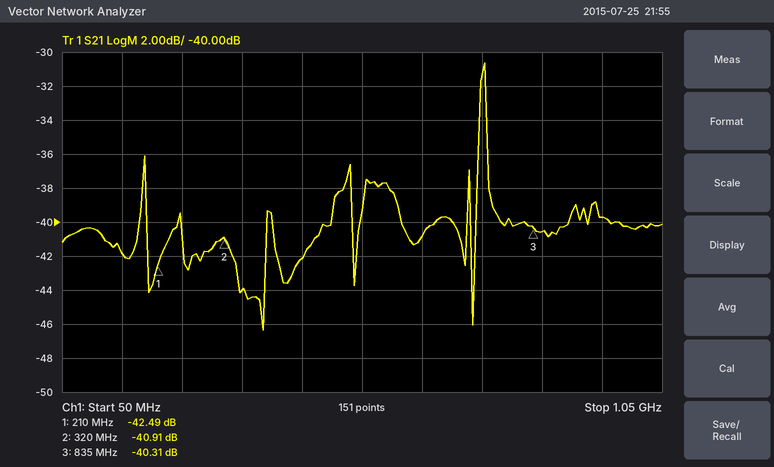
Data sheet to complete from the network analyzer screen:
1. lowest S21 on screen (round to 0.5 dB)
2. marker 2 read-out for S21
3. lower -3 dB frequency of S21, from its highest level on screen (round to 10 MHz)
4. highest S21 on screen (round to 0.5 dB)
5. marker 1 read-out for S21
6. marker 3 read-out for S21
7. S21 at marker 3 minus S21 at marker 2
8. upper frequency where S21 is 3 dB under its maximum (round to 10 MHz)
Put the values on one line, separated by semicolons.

-46.5 dB; -40.91 dB; 750 MHz; -30.5 dB; -42.49 dB; -40.31 dB; 0.60 dB; 760 MHz
